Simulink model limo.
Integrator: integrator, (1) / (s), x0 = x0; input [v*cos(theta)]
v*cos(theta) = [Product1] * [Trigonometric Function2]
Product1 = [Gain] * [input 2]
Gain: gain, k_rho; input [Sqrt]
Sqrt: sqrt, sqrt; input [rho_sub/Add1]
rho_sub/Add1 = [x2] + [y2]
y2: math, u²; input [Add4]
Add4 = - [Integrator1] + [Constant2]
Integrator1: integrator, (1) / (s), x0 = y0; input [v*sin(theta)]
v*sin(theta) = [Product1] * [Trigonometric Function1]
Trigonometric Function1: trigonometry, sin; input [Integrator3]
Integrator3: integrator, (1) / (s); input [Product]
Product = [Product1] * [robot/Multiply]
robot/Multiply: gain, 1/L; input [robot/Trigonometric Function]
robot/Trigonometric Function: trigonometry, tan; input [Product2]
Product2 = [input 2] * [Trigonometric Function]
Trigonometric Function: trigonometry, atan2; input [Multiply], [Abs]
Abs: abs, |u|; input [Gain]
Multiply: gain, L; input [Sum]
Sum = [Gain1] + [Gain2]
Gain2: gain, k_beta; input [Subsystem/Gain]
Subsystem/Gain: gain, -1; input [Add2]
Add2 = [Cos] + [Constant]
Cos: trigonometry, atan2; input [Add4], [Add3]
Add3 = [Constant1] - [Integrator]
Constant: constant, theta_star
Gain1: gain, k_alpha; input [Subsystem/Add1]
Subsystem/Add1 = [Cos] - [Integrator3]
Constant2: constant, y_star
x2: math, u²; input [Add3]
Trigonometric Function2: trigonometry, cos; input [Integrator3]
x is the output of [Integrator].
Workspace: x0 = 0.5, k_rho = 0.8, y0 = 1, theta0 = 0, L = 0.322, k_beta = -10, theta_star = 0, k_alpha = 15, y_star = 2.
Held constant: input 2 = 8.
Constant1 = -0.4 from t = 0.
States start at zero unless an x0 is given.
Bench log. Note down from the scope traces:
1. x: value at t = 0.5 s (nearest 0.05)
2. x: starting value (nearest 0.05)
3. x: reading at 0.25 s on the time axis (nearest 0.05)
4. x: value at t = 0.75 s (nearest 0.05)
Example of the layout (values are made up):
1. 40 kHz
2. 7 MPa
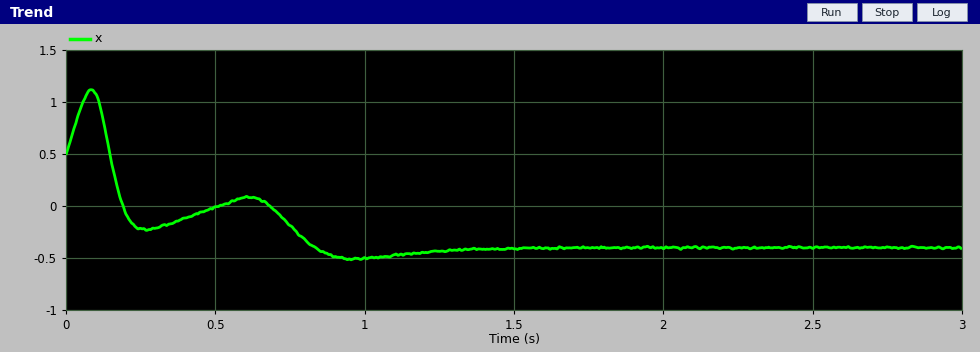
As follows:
1. 0.00
2. 0.50
3. -0.20
4. -0.20
